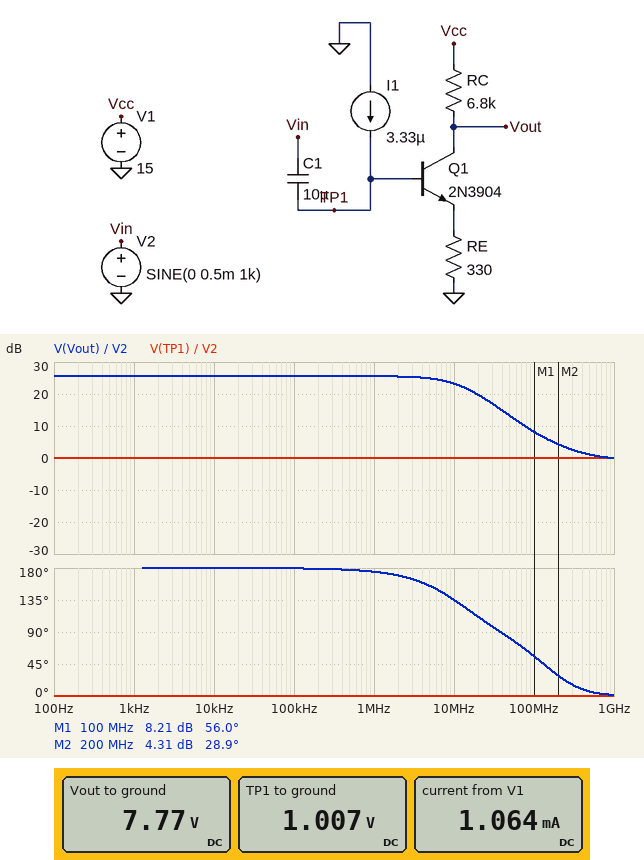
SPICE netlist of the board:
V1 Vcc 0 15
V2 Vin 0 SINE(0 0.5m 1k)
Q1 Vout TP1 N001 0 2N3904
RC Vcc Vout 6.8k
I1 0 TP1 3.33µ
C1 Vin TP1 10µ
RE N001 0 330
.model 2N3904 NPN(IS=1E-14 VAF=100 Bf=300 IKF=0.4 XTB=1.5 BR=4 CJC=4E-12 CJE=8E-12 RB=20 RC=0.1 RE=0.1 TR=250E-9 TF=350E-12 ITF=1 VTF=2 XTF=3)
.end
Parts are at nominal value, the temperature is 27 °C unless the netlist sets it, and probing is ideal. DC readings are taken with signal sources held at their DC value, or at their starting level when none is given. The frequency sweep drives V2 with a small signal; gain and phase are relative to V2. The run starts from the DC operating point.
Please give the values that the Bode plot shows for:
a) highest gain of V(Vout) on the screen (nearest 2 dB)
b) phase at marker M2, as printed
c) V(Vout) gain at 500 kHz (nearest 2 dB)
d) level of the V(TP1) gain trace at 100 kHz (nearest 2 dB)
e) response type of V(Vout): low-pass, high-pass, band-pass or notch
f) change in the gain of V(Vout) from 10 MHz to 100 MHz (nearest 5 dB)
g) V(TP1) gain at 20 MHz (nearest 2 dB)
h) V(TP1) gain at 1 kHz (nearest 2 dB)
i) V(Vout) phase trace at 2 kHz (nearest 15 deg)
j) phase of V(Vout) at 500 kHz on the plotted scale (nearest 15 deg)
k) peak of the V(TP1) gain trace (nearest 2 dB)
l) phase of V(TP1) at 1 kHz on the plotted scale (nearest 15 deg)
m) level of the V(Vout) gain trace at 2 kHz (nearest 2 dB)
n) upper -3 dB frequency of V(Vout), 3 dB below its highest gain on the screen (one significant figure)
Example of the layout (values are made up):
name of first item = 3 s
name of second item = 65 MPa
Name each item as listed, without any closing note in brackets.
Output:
highest gain of V(Vout) on the screen = 26 dB
phase at marker M2, as printed = 28.9 deg
V(Vout) gain at 500 kHz = 26 dB
level of the V(TP1) gain trace at 100 kHz = 0 dB
response type of V(Vout): low-pass, high-pass, band-pass or notch = low-pass
change in the gain of V(Vout) from 10 MHz to 100 MHz = -15 dB
V(TP1) gain at 20 MHz = 0 dB
V(TP1) gain at 1 kHz = 0 dB
V(Vout) phase trace at 2 kHz = 180 deg
phase of V(Vout) at 500 kHz on the plotted scale = 180 deg
peak of the V(TP1) gain trace = 0 dB
phase of V(TP1) at 1 kHz on the plotted scale = 0 deg
level of the V(Vout) gain trace at 2 kHz = 26 dB
upper -3 dB frequency of V(Vout), 3 dB below its highest gain on the screen = 10 MHz
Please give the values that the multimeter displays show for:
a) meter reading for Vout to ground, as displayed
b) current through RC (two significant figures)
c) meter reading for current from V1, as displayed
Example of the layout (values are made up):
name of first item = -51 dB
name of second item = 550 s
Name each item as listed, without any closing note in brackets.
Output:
meter reading for Vout to ground, as displayed = 7.77 V
current through RC = 1.1 mA
meter reading for current from V1, as displayed = 1.064 mA
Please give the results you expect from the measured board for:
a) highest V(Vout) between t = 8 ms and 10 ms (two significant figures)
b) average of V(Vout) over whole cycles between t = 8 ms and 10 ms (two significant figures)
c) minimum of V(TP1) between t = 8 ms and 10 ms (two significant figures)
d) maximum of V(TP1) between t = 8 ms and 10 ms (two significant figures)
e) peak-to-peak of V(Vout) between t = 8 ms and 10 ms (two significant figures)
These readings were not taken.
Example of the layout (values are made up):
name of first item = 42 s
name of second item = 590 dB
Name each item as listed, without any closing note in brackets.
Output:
highest V(Vout) between t = 8 ms and 10 ms = 7.8 V
average of V(Vout) over whole cycles between t = 8 ms and 10 ms = 7.8 V
minimum of V(TP1) between t = 8 ms and 10 ms = 1.0 V
maximum of V(TP1) between t = 8 ms and 10 ms = 1.0 V
peak-to-peak of V(Vout) between t = 8 ms and 10 ms = 19 mV
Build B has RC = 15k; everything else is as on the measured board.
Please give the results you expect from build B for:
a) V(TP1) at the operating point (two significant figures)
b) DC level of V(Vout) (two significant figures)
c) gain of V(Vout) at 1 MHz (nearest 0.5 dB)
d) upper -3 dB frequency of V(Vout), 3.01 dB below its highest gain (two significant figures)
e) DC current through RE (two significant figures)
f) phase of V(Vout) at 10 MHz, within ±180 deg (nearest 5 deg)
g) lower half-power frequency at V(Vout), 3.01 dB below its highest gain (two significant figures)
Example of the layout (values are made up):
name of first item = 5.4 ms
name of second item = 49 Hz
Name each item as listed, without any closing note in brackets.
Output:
V(TP1) at the operating point = 970 mV
DC level of V(Vout) = 520 mV
gain of V(Vout) at 1 MHz = 29.5 dB
upper -3 dB frequency of V(Vout), 3.01 dB below its highest gain = 1.2 MHz
DC current through RE = 970 µA
phase of V(Vout) at 10 MHz, within ±180 deg = 85 deg
lower half-power frequency at V(Vout), 3.01 dB below its highest gain = 2.4 Hz
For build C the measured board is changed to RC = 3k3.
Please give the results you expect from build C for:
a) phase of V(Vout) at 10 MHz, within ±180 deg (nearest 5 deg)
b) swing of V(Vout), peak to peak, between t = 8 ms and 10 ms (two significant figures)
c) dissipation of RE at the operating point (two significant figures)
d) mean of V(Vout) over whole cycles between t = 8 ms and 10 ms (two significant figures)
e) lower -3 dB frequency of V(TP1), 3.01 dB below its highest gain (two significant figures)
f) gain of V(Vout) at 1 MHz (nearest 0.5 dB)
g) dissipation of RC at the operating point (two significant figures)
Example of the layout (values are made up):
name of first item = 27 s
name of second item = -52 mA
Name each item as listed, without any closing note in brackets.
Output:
phase of V(Vout) at 10 MHz, within ±180 deg = 155 deg
swing of V(Vout), peak to peak, between t = 8 ms and 10 ms = 9.3 mV
dissipation of RE at the operating point = 400 µW
mean of V(Vout) over whole cycles between t = 8 ms and 10 ms = 11 V
lower -3 dB frequency of V(TP1), 3.01 dB below its highest gain = 140 mHz
gain of V(Vout) at 1 MHz = 19.5 dB
dissipation of RC at the operating point = 4.0 mW
